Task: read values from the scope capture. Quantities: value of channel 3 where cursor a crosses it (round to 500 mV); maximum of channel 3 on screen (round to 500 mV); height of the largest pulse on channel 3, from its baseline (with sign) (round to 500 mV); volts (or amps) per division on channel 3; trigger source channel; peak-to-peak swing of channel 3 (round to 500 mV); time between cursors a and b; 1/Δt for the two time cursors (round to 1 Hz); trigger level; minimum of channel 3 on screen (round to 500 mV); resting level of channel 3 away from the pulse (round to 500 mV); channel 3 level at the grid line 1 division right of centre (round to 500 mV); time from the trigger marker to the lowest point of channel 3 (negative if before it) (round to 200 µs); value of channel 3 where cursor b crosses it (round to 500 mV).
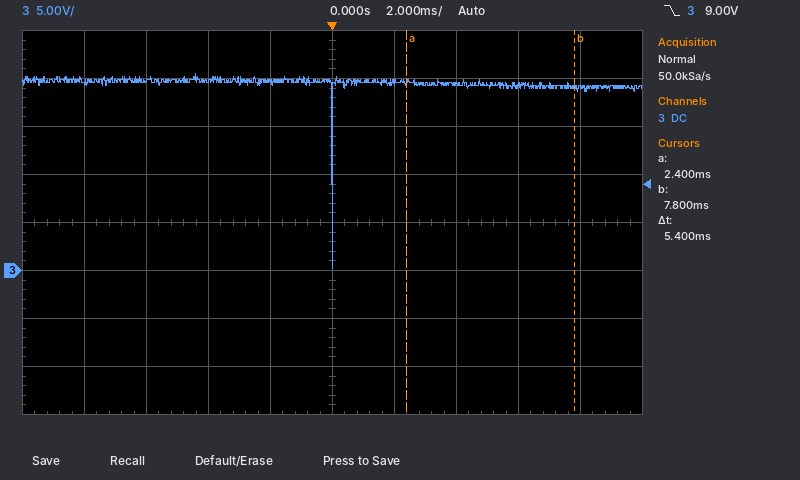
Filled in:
19.5 V
20.5 V
-19.5 V
5 V
channel 3
20.5 V
5.4 ms
185 Hz
9.00 V
0.0 V
19.5 V
19.5 V
0.0 ms
19.0 V
